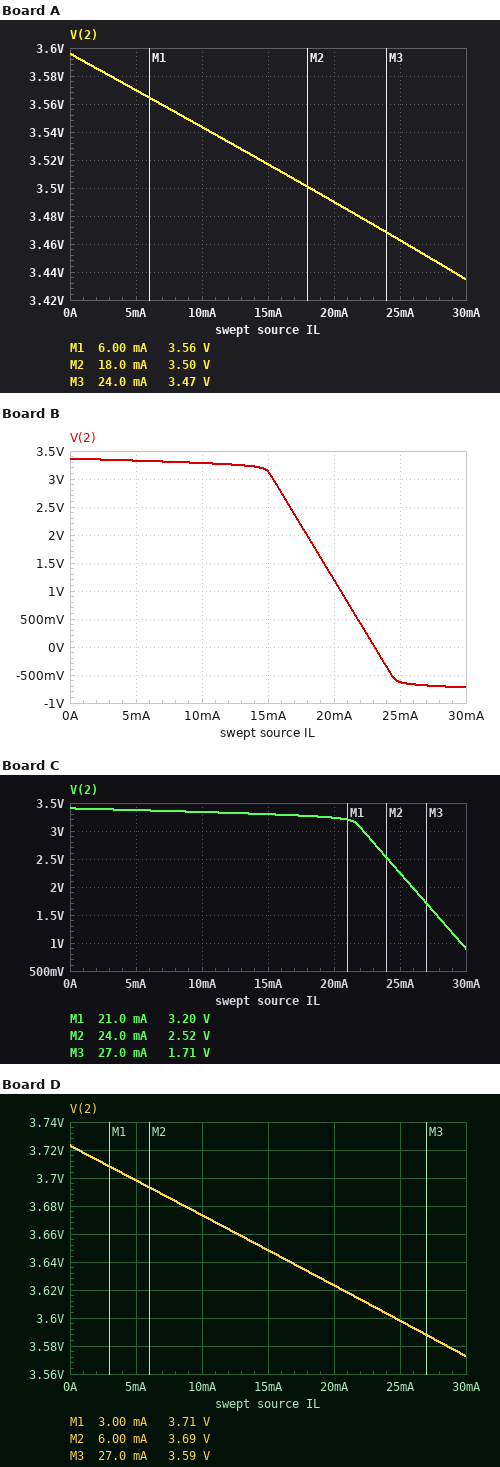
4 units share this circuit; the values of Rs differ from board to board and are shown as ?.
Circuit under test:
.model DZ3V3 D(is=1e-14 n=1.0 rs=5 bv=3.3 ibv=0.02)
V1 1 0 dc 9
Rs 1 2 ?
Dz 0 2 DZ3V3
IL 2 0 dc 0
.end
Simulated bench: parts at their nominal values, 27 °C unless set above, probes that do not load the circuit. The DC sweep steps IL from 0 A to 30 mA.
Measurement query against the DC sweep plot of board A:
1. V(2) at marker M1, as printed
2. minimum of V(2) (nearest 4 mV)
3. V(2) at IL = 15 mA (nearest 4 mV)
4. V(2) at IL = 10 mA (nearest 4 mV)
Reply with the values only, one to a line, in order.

3.56 V
3.436 V
3.516 V
3.544 V
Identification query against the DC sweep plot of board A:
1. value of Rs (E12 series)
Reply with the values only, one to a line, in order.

100 Ω
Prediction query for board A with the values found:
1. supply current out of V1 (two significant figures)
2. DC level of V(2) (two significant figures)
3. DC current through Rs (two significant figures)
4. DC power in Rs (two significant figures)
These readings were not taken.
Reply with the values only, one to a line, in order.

54 mA
3.6 V
54 mA
290 mW
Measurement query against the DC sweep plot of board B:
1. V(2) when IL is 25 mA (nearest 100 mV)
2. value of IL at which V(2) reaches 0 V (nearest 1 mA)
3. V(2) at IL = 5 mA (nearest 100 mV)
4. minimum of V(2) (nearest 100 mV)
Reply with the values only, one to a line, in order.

-600 mV
23 mA
3.3 V
-700 mV
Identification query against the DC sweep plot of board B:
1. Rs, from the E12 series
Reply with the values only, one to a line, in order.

390 Ω
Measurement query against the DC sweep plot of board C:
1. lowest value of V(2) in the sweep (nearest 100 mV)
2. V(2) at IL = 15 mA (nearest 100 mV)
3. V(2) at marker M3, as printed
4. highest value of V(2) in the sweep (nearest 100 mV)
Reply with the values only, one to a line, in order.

900 mV
3.3 V
1.71 V
3.4 V
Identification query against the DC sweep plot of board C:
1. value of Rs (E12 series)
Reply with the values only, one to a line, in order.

270 Ω
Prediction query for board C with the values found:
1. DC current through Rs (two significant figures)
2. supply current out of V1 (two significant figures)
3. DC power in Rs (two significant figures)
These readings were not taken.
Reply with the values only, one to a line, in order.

21 mA
21 mA
120 mW
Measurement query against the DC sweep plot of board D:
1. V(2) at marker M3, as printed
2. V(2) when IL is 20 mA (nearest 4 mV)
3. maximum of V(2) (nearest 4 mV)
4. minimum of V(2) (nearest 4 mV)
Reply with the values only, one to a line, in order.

3.59 V
3.624 V
3.724 V
3.572 V
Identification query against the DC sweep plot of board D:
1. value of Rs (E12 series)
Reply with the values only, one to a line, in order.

68 Ω
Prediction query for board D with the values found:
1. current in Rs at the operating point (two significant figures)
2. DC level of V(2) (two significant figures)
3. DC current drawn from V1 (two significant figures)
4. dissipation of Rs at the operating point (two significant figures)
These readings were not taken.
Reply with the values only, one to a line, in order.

78 mA
3.7 V
78 mA
410 mW
